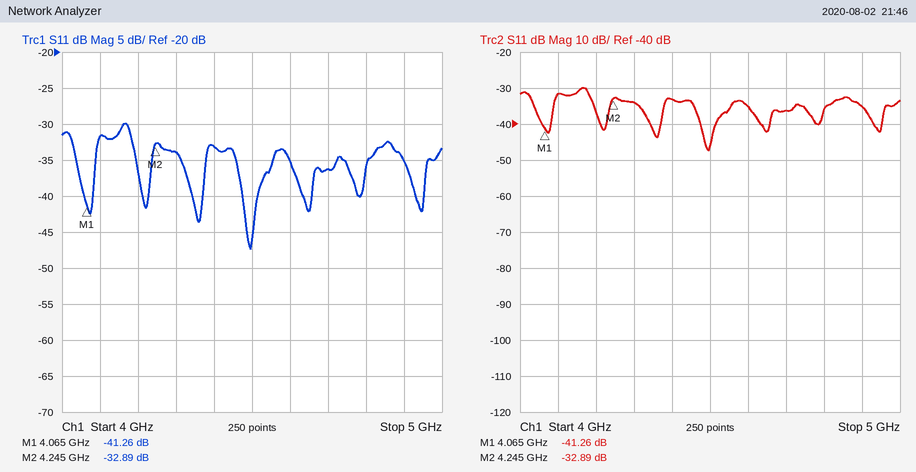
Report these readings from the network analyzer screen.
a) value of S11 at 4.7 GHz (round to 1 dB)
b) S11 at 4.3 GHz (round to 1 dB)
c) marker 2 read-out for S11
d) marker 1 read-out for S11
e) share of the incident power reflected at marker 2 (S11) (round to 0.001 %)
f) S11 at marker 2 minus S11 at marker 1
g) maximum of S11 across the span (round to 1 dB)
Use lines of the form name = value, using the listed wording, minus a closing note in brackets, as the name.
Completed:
value of S11 at 4.7 GHz = -36 dB
S11 at 4.3 GHz = -34 dB
marker 2 read-out for S11 = -32.89 dB
marker 1 read-out for S11 = -41.26 dB
share of the incident power reflected at marker 2 (S11) = 0.051 %
S11 at marker 2 minus S11 at marker 1 = 8.37 dB
maximum of S11 across the span = -30 dB
